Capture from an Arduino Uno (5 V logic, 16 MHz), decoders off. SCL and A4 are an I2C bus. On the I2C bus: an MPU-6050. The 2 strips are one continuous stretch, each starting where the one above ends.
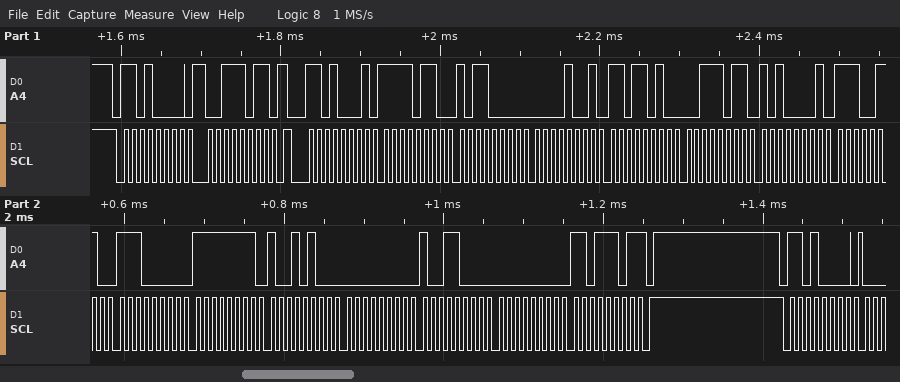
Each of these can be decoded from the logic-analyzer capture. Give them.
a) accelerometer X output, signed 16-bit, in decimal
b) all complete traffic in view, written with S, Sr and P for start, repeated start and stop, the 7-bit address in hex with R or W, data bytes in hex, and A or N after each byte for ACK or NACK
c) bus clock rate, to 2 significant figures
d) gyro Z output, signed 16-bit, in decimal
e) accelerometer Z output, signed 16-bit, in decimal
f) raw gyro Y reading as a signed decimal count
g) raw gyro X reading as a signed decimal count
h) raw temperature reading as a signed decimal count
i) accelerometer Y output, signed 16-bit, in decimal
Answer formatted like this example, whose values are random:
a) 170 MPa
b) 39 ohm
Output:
a) -2384
b) S 68W A 3B A Sr 68R A F6 A B0 A 09 A DA A 3B A A1 A E6 A E0 A FF A 94 A 00 A 98 A 00 A DD N P S 68W A
c) 100 kHz
d) 221
e) 15265
f) 152
g) -108
h) -6432
i) 2522
